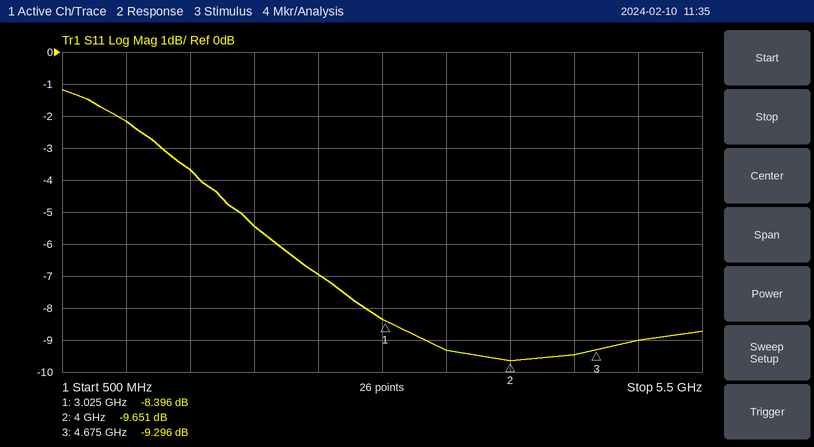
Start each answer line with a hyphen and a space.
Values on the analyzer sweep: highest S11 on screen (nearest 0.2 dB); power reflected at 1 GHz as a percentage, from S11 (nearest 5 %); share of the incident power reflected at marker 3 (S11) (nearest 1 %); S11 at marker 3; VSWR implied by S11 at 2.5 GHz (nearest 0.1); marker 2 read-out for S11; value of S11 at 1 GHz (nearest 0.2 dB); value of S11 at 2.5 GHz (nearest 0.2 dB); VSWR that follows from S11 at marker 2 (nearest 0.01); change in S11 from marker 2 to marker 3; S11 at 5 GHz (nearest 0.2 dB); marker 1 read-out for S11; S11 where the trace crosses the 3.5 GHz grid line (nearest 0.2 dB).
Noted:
- -1.2 dB
- 60 %
- 12 %
- -9.296 dB
- 2.6
- -9.651 dB
- -2.2 dB
- -7.0 dB
- 1.98
- 0.355 dB
- -9.0 dB
- -8.396 dB
- -9.4 dB
